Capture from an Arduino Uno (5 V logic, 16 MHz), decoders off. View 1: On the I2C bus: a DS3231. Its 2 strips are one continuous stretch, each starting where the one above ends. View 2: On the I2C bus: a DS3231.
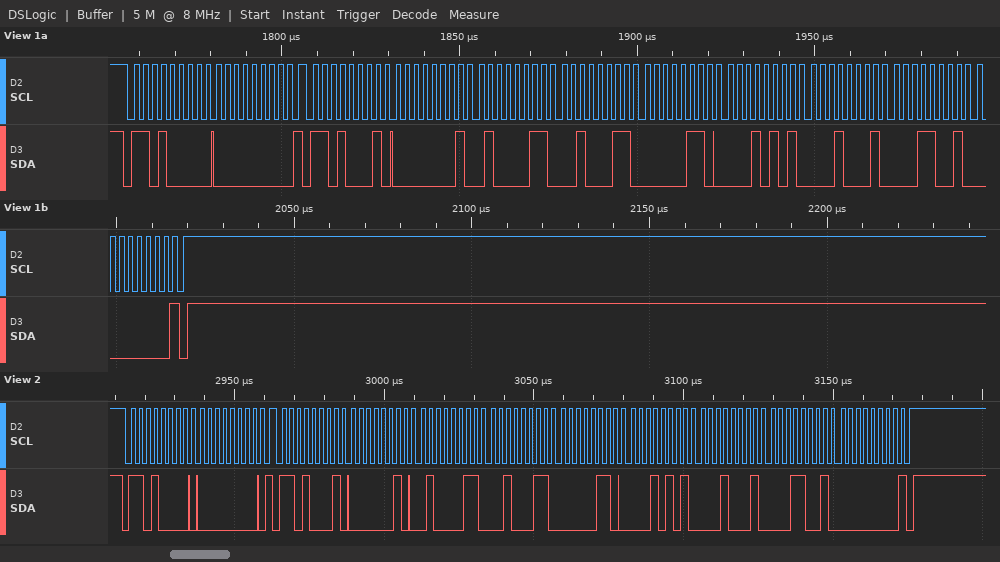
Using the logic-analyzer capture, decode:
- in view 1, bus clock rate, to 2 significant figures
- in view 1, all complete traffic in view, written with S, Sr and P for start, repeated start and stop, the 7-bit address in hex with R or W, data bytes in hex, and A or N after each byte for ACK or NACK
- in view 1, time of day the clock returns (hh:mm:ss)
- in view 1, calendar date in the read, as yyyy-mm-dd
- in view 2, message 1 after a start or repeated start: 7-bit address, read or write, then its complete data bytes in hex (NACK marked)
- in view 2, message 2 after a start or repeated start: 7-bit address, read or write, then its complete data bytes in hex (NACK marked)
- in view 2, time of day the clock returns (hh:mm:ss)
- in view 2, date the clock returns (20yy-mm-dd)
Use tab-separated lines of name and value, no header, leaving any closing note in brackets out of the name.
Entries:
in view 1, bus clock rate, to 2 significant figures	400 kHz
in view 1, all complete traffic in view, written with S, Sr and P for start, repeated start and stop, the 7-bit address in hex with R or W, data bytes in hex, and A or N after each byte for ACK or NACK	S 68W A 00 A Sr 68R A 01 A 43 A 23 A 06 A 15 A 11 A 19 A 00 N P
in view 1, time of day the clock returns	23:43:01
in view 1, calendar date in the read, as yyyy-mm-dd	2019-11-15
in view 2, message 1 after a start or repeated start: 7-bit address, read or write, then its complete data bytes in hex	0x68 write: 00
in view 2, message 2 after a start or repeated start: 7-bit address, read or write, then its complete data bytes in hex	0x68 read: 02 43 23 06 15 11 19 00 NACK
in view 2, time of day the clock returns	23:43:02
in view 2, date the clock returns	2019-11-15
